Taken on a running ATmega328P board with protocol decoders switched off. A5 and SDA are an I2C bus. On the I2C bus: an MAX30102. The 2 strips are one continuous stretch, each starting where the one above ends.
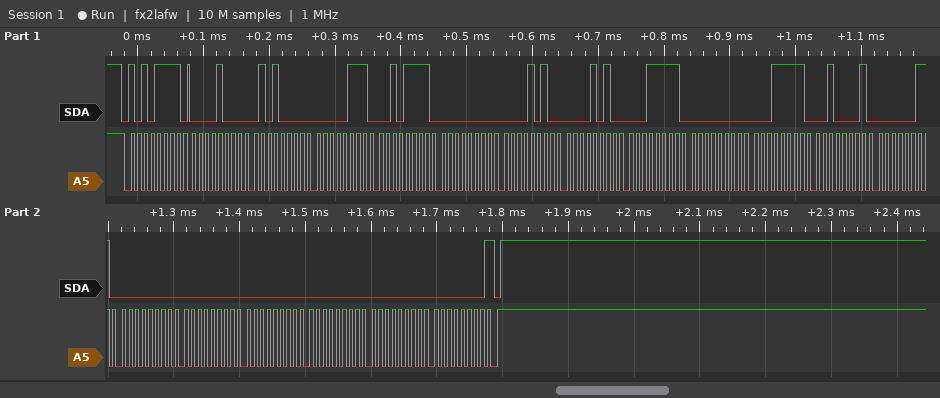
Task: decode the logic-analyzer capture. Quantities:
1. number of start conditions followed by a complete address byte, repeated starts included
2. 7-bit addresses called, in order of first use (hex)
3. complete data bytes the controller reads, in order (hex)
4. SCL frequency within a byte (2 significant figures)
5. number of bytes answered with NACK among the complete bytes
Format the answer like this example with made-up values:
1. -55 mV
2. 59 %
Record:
1. 1
2. 0x57
3. 08 50 07 2F 00 0A 0A 1F 00 1F 21 03 00 00 00 00 00 00
4. 100 kHz
5. 1
